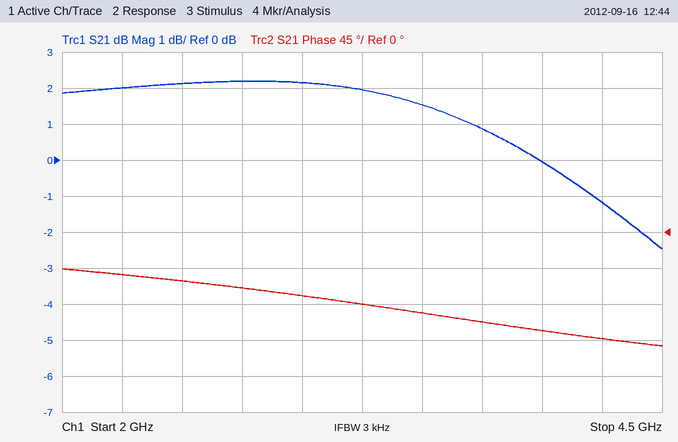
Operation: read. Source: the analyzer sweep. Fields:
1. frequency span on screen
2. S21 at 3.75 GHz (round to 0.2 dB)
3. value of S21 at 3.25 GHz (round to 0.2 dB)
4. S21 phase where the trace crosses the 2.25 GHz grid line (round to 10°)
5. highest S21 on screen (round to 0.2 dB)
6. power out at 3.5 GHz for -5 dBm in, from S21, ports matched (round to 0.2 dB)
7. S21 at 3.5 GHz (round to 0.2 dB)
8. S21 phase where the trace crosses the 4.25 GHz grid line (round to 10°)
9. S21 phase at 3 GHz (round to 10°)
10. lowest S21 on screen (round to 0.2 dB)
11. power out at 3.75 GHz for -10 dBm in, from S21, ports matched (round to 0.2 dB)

2.5 GHz
0.8 dB
2.0 dB
-50°
2.2 dB
-3.4 dBm
1.6 dB
-130°
-80°
-2.4 dB
-9.2 dBm
